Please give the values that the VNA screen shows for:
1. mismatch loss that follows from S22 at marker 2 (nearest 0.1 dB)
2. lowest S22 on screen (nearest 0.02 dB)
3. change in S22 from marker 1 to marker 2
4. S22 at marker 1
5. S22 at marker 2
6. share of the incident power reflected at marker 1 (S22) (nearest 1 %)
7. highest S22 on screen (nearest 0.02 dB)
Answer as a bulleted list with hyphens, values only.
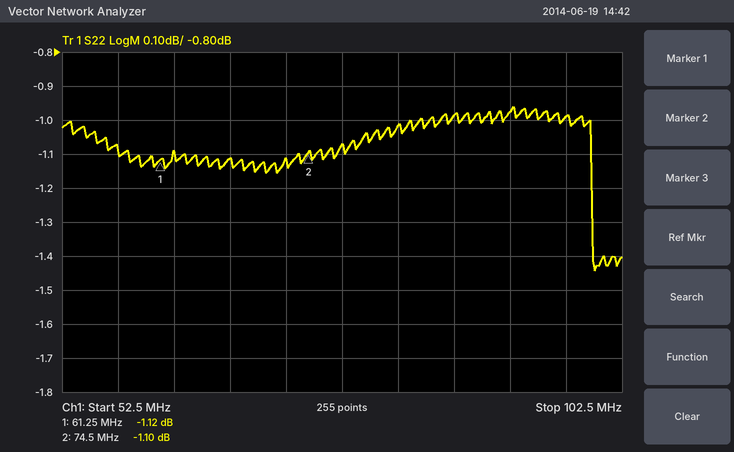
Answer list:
- 6.5 dB
- -1.44 dB
- 0.02 dB
- -1.12 dB
- -1.10 dB
- 77 %
- -0.96 dB
